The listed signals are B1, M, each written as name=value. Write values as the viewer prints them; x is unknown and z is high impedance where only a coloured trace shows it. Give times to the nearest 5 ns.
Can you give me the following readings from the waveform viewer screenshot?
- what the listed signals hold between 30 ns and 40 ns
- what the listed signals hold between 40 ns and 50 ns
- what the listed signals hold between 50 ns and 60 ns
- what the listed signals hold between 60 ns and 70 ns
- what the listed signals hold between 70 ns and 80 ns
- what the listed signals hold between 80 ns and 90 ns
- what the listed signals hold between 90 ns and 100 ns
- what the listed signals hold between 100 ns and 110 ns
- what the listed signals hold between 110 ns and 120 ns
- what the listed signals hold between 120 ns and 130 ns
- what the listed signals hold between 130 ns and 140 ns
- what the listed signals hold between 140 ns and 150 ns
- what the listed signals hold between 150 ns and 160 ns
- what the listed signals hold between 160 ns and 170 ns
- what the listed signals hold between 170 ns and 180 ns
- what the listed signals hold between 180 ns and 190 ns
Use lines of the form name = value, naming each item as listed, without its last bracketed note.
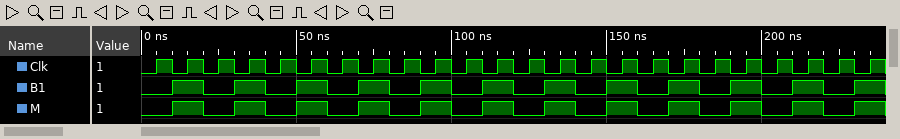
what the listed signals hold between 30 ns and 40 ns = B1=1, M=1
what the listed signals hold between 40 ns and 50 ns = B1=0, M=0
what the listed signals hold between 50 ns and 60 ns = B1=1, M=1
what the listed signals hold between 60 ns and 70 ns = B1=0, M=0
what the listed signals hold between 70 ns and 80 ns = B1=1, M=1
what the listed signals hold between 80 ns and 90 ns = B1=0, M=0
what the listed signals hold between 90 ns and 100 ns = B1=1, M=1
what the listed signals hold between 100 ns and 110 ns = B1=0, M=0
what the listed signals hold between 110 ns and 120 ns = B1=1, M=1
what the listed signals hold between 120 ns and 130 ns = B1=0, M=0
what the listed signals hold between 130 ns and 140 ns = B1=1, M=1
what the listed signals hold between 140 ns and 150 ns = B1=0, M=0
what the listed signals hold between 150 ns and 160 ns = B1=1, M=1
what the listed signals hold between 160 ns and 170 ns = B1=0, M=0
what the listed signals hold between 170 ns and 180 ns = B1=1, M=1
what the listed signals hold between 180 ns and 190 ns = B1=0, M=0
